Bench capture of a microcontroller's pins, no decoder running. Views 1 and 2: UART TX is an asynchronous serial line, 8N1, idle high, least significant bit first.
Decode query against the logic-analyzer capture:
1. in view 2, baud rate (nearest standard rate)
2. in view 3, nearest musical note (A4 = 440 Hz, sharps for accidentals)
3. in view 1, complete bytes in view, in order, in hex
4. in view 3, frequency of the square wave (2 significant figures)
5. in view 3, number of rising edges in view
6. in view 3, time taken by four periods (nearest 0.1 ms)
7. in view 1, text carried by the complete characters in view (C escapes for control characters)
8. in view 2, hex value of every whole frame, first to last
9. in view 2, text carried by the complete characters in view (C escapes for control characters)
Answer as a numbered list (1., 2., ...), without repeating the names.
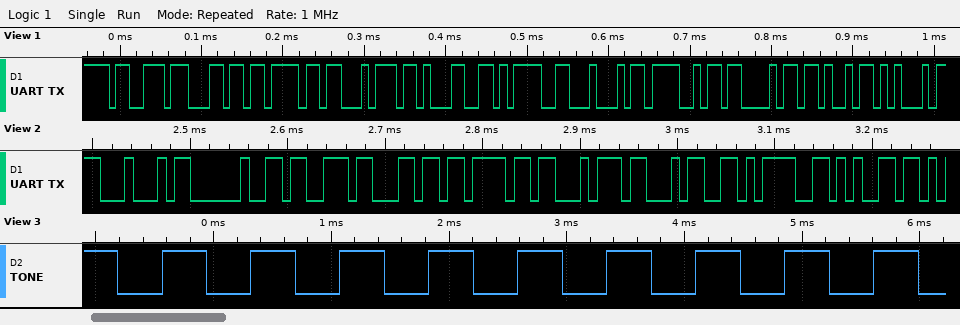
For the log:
1. 115200 baud
2. E6
3. 73 6C 6F 74 31 3D 44 4F 43 4B 45
4. 1.3 kHz
5. 9
6. 3.0 ms
7. "slot1=DOCKE"
8. 44 20 73 6C 6F 74 34 3D 65
9. "D slot4=e"
